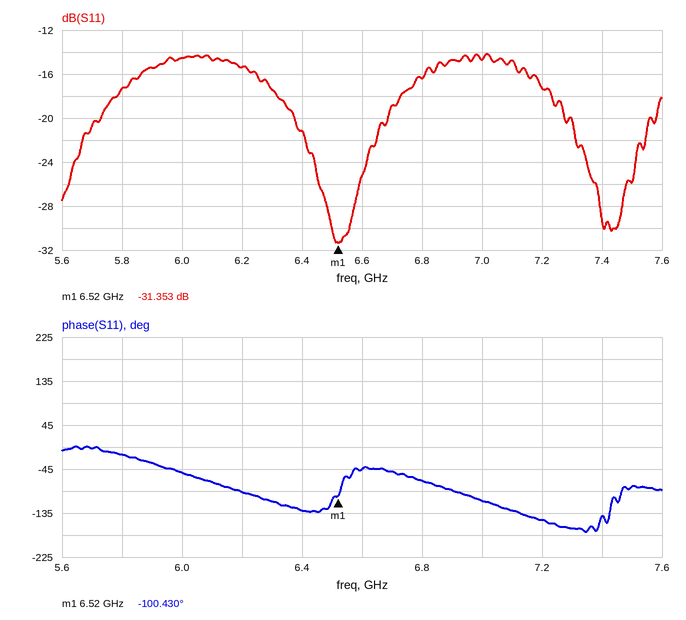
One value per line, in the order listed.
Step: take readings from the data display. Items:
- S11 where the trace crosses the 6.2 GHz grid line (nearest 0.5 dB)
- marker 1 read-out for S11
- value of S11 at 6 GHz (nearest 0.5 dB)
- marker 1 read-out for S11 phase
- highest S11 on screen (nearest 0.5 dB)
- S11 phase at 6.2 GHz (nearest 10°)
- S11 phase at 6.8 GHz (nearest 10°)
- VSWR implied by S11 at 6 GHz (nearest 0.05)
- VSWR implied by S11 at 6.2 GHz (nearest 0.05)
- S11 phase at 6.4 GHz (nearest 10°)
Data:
-15.5 dB
-31.353 dB
-14.5 dB
-100.430°
-14.0 dB
-90°
-70°
1.45
1.40
-130°
